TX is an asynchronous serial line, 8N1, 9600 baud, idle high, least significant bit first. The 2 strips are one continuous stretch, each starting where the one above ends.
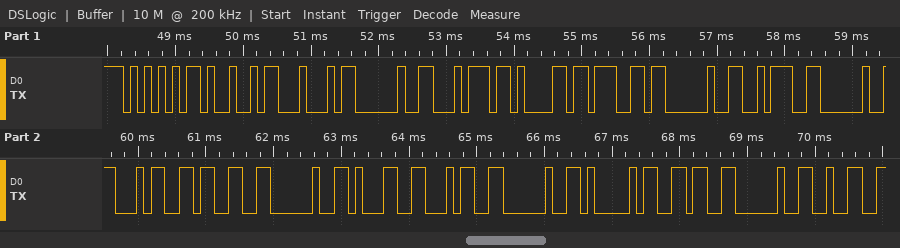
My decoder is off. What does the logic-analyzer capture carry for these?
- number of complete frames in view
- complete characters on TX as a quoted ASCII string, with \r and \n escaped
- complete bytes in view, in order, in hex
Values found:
20
"UID tag : 43 14 A6 2"
55 49 44 20 74 61 67 20 3A 20 34 33 20 31 34 20 41 36 20 32
